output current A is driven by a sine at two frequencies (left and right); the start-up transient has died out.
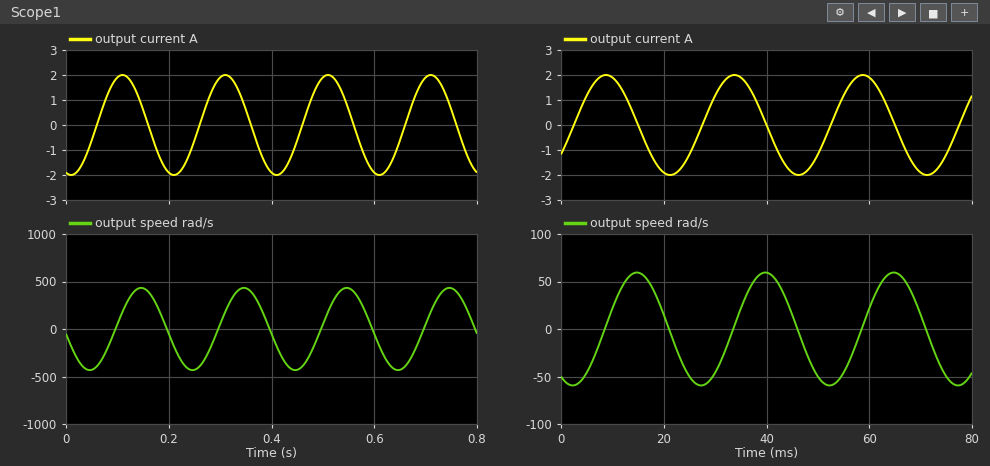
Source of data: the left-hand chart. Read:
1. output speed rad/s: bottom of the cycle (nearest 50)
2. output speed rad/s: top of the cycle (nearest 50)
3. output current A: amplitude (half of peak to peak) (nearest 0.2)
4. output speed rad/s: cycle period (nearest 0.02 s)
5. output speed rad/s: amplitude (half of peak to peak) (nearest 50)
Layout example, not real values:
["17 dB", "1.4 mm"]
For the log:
["-450", "450", "2.0", "0.20 s", "450"]
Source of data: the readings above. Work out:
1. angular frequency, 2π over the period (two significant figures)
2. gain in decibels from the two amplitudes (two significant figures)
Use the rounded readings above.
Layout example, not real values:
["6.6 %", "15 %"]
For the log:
["31 rad/s", "47 dB"]
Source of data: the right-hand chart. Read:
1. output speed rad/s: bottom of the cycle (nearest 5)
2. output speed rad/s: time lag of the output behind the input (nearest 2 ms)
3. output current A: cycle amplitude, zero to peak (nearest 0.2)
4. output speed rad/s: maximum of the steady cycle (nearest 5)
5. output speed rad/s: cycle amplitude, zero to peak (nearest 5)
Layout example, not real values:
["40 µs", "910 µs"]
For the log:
["-60", "6 ms", "2.0", "60", "60"]
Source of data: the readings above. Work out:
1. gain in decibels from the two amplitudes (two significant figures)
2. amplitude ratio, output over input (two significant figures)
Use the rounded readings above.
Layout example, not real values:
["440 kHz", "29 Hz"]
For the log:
["30 dB", "30"]
